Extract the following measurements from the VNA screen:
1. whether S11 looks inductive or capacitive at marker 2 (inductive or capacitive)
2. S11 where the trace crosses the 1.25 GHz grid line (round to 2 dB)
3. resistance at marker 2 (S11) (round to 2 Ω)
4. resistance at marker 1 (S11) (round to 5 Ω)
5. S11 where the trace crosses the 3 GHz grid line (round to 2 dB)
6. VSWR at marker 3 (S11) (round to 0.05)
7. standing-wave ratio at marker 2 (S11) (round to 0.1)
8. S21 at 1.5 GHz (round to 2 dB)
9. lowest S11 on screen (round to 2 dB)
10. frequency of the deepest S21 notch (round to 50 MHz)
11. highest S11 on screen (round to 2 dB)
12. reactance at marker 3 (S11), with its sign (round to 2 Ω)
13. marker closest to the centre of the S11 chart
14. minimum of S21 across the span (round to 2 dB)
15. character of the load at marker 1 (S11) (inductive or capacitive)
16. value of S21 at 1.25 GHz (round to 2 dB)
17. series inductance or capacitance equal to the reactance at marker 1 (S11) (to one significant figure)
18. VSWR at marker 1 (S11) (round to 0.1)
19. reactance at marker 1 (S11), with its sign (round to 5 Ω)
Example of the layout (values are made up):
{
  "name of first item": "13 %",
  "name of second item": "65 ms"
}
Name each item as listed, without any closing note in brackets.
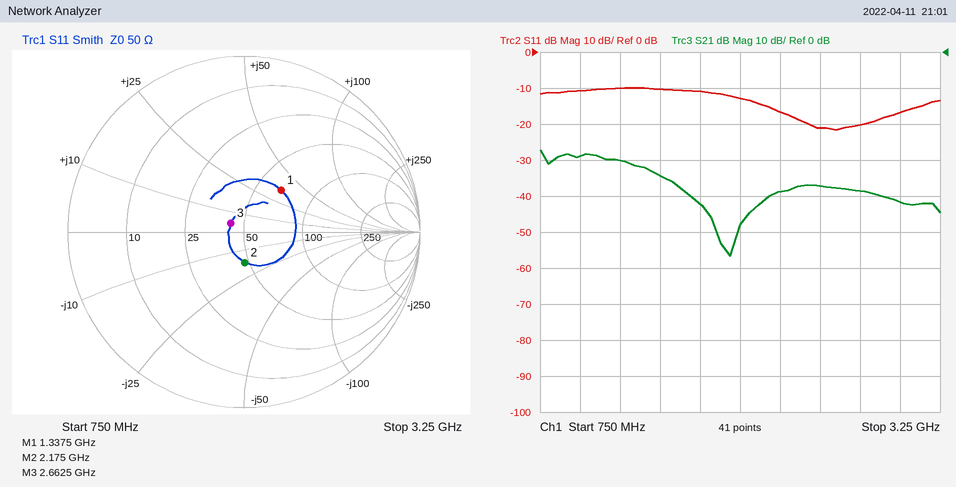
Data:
{
  "whether S11 looks inductive or capacitive at marker 2": "capacitive",
  "S11 where the trace crosses the 1.25 GHz grid line": "-10 dB",
  "resistance at marker 2 (S11)": "48 Ω",
  "resistance at marker 1 (S11)": "65 Ω",
  "S11 where the trace crosses the 3 GHz grid line": "-16 dB",
  "VSWR at marker 3 (S11)": "1.20",
  "standing-wave ratio at marker 2 (S11)": "1.4",
  "S21 at 1.5 GHz": "-34 dB",
  "lowest S11 on screen": "-22 dB",
  "frequency of the deepest S21 notch": "1.95 GHz",
  "highest S11 on screen": "-10 dB",
  "reactance at marker 3 (S11), with its sign": "+4 Ω",
  "marker closest to the centre of the S11 chart": "marker 3",
  "minimum of S21 across the span": "-56 dB",
  "character of the load at marker 1 (S11)": "inductive",
  "value of S21 at 1.25 GHz": "-30 dB",
  "series inductance or capacitance equal to the reactance at marker 1 (S11)": "4 nH",
  "VSWR at marker 1 (S11)": "1.9",
  "reactance at marker 1 (S11), with its sign": "+35 Ω"
}
